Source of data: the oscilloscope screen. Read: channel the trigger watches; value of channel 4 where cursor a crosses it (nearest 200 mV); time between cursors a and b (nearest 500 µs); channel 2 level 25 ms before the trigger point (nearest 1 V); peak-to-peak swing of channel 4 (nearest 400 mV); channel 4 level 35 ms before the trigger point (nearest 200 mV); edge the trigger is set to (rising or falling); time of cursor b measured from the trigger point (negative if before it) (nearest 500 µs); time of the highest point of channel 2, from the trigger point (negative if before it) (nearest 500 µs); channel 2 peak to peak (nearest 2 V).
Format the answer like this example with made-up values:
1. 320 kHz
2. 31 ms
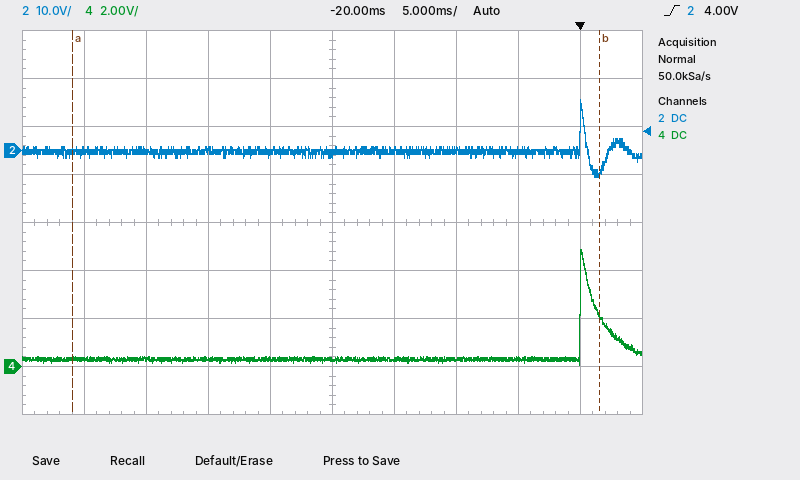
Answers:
1. channel 2
2. 400 mV
3. 42.5 ms
4. -1 V
5. 4.8 V
6. 400 mV
7. rising
8. +1.5 ms
9. 0.0 ms
10. 16 V
